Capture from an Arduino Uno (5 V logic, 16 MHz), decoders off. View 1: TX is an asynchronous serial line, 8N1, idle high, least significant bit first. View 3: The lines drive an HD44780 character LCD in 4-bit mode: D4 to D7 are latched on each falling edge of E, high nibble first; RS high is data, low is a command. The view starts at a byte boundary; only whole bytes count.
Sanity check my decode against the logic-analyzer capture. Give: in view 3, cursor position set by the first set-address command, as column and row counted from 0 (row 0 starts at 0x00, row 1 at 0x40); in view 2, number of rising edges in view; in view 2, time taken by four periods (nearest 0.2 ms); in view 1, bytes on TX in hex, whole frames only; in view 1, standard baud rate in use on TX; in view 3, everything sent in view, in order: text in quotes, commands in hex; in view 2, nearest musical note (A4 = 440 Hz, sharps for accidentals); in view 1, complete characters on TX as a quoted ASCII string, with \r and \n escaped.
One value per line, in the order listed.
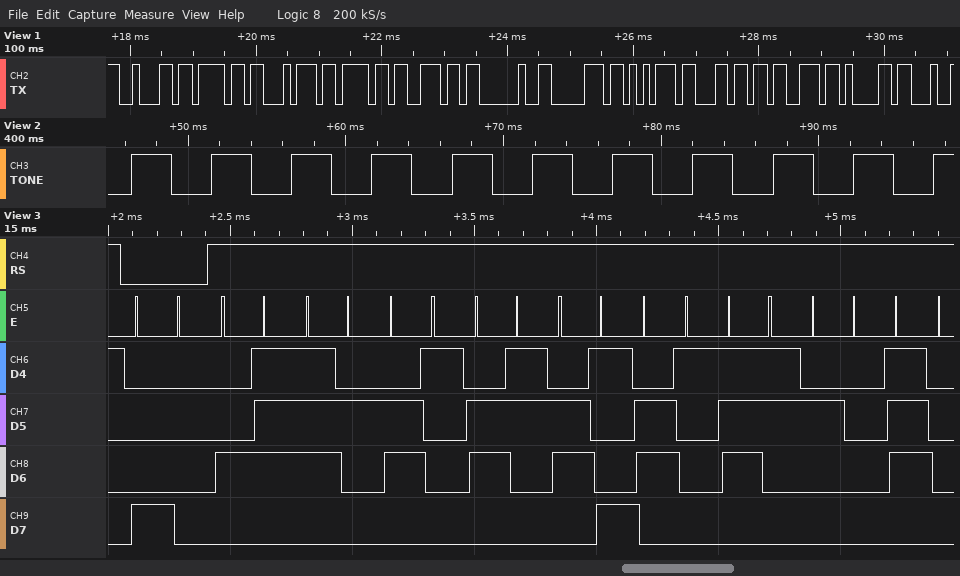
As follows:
column 0, row 0
11
20.4 ms
62 6F 74 6F 6E 20 70 75 6C 73 61
9600 baud
0x80 "Gracias p"
G3
"boton pulsa"
